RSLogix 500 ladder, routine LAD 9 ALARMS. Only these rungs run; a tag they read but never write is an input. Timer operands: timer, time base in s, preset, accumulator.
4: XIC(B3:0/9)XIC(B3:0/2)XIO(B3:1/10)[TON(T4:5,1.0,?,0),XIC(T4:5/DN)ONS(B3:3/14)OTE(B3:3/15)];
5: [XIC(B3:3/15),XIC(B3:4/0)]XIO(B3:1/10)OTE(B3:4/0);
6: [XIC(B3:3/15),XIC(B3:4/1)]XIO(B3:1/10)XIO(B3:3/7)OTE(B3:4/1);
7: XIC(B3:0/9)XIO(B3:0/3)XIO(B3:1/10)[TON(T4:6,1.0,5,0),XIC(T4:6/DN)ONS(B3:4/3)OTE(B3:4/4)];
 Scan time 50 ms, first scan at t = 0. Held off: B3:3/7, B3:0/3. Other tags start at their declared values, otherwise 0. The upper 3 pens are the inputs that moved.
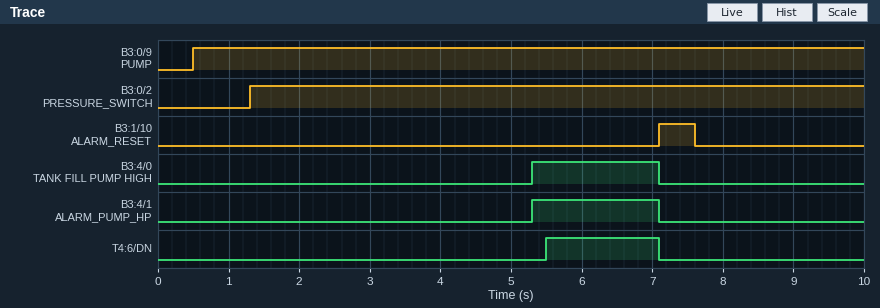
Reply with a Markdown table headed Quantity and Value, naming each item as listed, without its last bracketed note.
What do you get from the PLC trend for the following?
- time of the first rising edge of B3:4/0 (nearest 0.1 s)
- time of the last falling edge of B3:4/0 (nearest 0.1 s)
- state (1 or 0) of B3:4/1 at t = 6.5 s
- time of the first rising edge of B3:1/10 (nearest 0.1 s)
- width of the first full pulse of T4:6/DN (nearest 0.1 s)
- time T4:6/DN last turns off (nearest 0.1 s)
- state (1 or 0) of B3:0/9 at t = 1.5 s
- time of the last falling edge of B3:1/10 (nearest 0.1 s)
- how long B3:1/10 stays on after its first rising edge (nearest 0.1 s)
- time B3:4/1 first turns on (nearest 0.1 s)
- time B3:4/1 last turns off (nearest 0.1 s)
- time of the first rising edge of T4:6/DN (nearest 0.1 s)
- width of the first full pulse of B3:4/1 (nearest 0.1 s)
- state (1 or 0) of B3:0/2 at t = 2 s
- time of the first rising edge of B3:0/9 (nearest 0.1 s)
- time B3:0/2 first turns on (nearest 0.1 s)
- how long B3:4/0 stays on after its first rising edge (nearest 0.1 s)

| Quantity | Value |
|---|---|
| time of the first rising edge of B3:4/0 | 5.3 s |
| time of the last falling edge of B3:4/0 | 7.1 s |
| state (1 or 0) of B3:4/1 at t = 6.5 s | 1 |
| time of the first rising edge of B3:1/10 | 7.1 s |
| width of the first full pulse of T4:6/DN | 1.6 s |
| time T4:6/DN last turns off | 7.1 s |
| state (1 or 0) of B3:0/9 at t = 1.5 s | 1 |
| time of the last falling edge of B3:1/10 | 7.6 s |
| how long B3:1/10 stays on after its first rising edge | 0.5 s |
| time B3:4/1 first turns on | 5.3 s |
| time B3:4/1 last turns off | 7.1 s |
| time of the first rising edge of T4:6/DN | 5.5 s |
| width of the first full pulse of B3:4/1 | 1.8 s |
| state (1 or 0) of B3:0/2 at t = 2 s | 1 |
| time of the first rising edge of B3:0/9 | 0.5 s |
| time B3:0/2 first turns on | 1.3 s |
| how long B3:4/0 stays on after its first rising edge | 1.8 s |
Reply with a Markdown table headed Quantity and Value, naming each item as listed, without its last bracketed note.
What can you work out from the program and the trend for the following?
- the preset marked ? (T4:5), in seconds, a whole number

| Quantity | Value |
|---|---|
| the preset marked ? (T4:5), in seconds, a whole number | 4 s |
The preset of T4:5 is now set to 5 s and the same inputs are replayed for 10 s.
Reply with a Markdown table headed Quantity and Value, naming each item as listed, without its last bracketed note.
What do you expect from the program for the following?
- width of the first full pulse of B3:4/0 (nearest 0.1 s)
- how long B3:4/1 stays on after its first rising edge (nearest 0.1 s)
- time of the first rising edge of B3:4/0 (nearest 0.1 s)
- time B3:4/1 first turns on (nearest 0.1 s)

| Quantity | Value |
|---|---|
| width of the first full pulse of B3:4/0 | 0.8 s |
| how long B3:4/1 stays on after its first rising edge | 0.8 s |
| time of the first rising edge of B3:4/0 | 6.3 s |
| time B3:4/1 first turns on | 6.3 s |
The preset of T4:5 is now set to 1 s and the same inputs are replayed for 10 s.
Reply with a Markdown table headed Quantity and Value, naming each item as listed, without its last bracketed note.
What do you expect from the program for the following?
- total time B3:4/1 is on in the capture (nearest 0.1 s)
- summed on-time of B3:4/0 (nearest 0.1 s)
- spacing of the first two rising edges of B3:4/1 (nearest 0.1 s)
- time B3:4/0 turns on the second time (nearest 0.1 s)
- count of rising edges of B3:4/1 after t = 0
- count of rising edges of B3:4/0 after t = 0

| Quantity | Value |
|---|---|
| total time B3:4/1 is on in the capture | 6.2 s |
| summed on-time of B3:4/0 | 6.2 s |
| spacing of the first two rising edges of B3:4/1 | 6.3 s |
| time B3:4/0 turns on the second time | 8.6 s |
| count of rising edges of B3:4/1 after t = 0 | 2 |
| count of rising edges of B3:4/0 after t = 0 | 2 |
